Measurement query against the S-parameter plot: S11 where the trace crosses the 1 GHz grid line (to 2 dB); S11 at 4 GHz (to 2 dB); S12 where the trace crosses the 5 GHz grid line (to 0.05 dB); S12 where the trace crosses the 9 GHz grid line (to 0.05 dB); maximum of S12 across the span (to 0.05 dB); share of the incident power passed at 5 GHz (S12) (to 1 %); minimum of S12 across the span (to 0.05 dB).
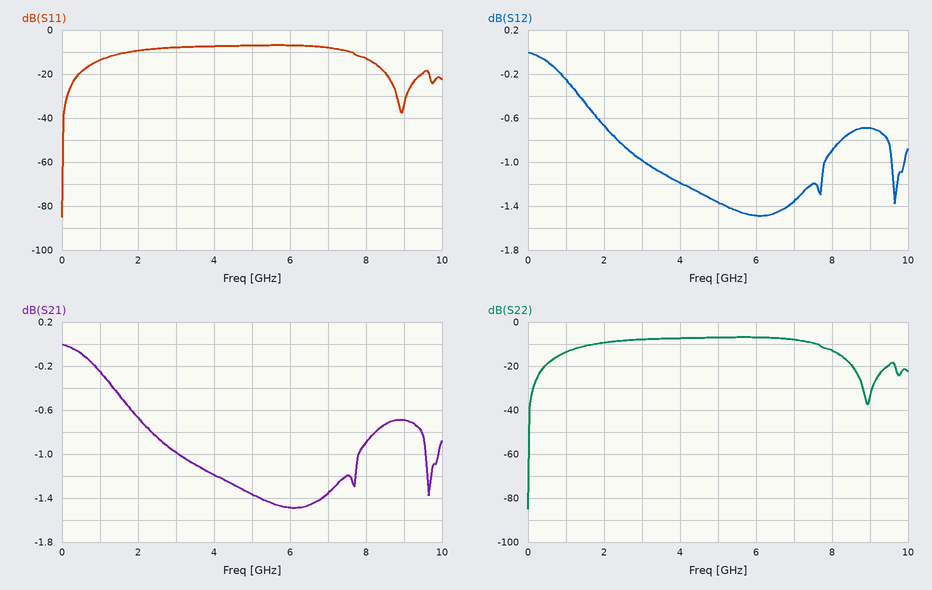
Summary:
-14 dB
-8 dB
-1.35 dB
-0.70 dB
0.00 dB
73 %
-1.50 dB
